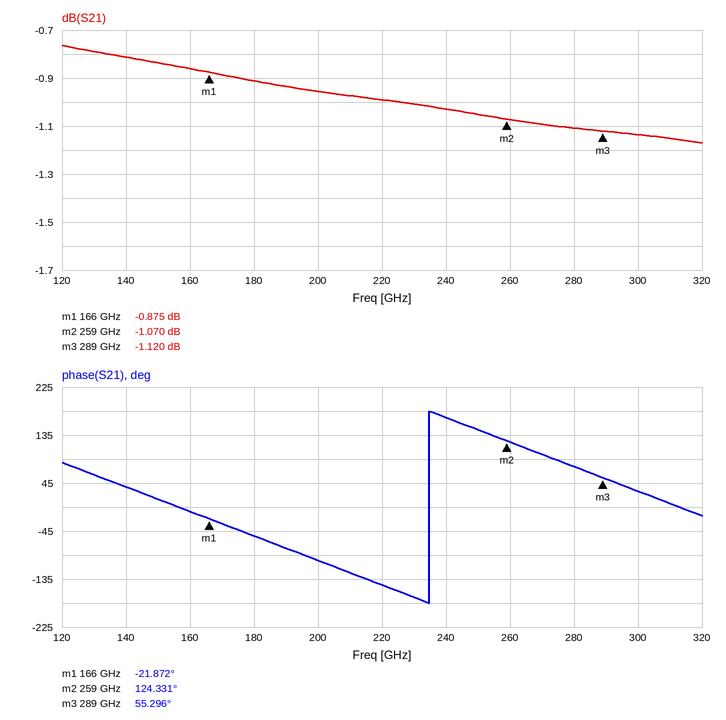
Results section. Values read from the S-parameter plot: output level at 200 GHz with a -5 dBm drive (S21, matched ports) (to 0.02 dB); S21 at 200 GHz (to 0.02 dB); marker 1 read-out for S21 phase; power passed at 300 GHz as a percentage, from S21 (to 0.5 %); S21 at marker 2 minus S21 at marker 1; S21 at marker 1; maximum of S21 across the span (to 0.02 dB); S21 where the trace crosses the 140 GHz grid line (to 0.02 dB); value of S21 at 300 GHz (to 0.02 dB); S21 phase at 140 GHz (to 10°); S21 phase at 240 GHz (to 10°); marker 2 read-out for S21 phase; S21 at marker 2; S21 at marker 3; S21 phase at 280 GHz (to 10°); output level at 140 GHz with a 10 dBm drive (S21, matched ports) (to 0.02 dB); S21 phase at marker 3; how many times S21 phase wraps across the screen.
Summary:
-5.96 dBm
-0.96 dB
-21.872°
77.0 %
-0.195 dB
-0.875 dB
-0.76 dB
-0.82 dB
-1.14 dB
40°
170°
124.331°
-1.070 dB
-1.120 dB
80°
9.18 dBm
55.296°
1
